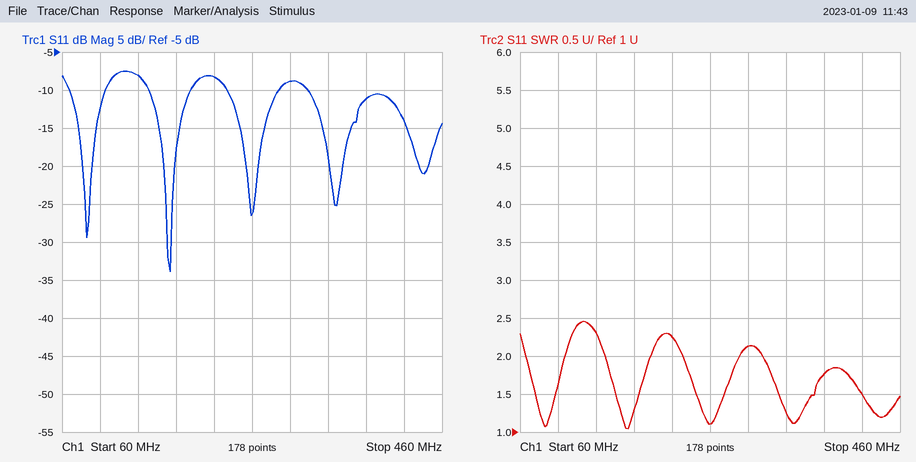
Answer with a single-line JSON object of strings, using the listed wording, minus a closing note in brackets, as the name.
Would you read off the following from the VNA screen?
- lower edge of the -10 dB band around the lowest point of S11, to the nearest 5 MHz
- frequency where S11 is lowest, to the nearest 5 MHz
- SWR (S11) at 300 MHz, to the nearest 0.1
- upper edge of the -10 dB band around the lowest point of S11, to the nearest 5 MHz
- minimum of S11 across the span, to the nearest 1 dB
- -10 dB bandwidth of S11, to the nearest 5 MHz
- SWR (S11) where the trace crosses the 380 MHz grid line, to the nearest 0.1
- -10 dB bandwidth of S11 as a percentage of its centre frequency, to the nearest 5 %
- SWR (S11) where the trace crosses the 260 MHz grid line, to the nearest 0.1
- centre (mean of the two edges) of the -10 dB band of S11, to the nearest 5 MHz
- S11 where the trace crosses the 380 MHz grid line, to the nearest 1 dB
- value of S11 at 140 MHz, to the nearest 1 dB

{"lower edge of the -10 dB band around the lowest point of S11, to the nearest 5 MHz": "150 MHz", "frequency where S11 is lowest, to the nearest 5 MHz": "175 MHz", "SWR (S11) at 300 MHz, to the nearest 0.1": "2.1", "upper edge of the -10 dB band around the lowest point of S11, to the nearest 5 MHz": "195 MHz", "minimum of S11 across the span, to the nearest 1 dB": "-34 dB", "-10 dB bandwidth of S11, to the nearest 5 MHz": "45 MHz", "SWR (S11) where the trace crosses the 380 MHz grid line, to the nearest 0.1": "1.8", "-10 dB bandwidth of S11 as a percentage of its centre frequency, to the nearest 5 %": "25 %", "SWR (S11) where the trace crosses the 260 MHz grid line, to the nearest 0.1": "1.1", "centre (mean of the two edges) of the -10 dB band of S11, to the nearest 5 MHz": "175 MHz", "S11 where the trace crosses the 380 MHz grid line, to the nearest 1 dB": "-11 dB", "value of S11 at 140 MHz, to the nearest 1 dB": "-8 dB"}
